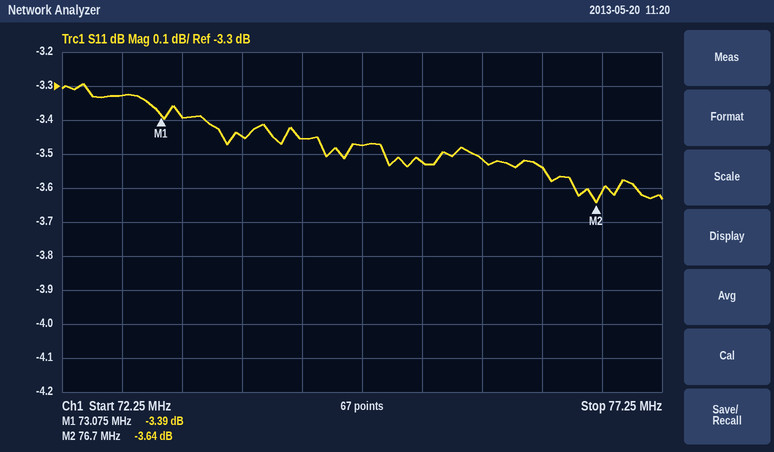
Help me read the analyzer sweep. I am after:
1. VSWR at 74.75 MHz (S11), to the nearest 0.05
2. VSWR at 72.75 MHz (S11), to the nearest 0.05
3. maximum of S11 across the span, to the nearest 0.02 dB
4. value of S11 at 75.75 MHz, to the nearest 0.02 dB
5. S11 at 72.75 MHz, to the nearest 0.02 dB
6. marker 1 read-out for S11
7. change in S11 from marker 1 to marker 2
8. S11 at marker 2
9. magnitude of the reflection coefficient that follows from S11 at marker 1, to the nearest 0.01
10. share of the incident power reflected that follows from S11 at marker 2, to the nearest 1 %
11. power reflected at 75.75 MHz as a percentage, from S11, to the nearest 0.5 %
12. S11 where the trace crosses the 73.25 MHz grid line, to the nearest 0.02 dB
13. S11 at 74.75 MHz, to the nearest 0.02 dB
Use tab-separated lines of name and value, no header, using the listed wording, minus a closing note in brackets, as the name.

VSWR at 74.75 MHz (S11), to the nearest 0.05	5.05
VSWR at 72.75 MHz (S11), to the nearest 0.05	5.30
maximum of S11 across the span, to the nearest 0.02 dB	-3.30 dB
value of S11 at 75.75 MHz, to the nearest 0.02 dB	-3.52 dB
S11 at 72.75 MHz, to the nearest 0.02 dB	-3.32 dB
marker 1 read-out for S11	-3.39 dB
change in S11 from marker 1 to marker 2	-0.25 dB
S11 at marker 2	-3.64 dB
magnitude of the reflection coefficient that follows from S11 at marker 1, to the nearest 0.01	0.68
share of the incident power reflected that follows from S11 at marker 2, to the nearest 1 %	43 %
power reflected at 75.75 MHz as a percentage, from S11, to the nearest 0.5 %	44.5 %
S11 where the trace crosses the 73.25 MHz grid line, to the nearest 0.02 dB	-3.40 dB
S11 at 74.75 MHz, to the nearest 0.02 dB	-3.48 dB
